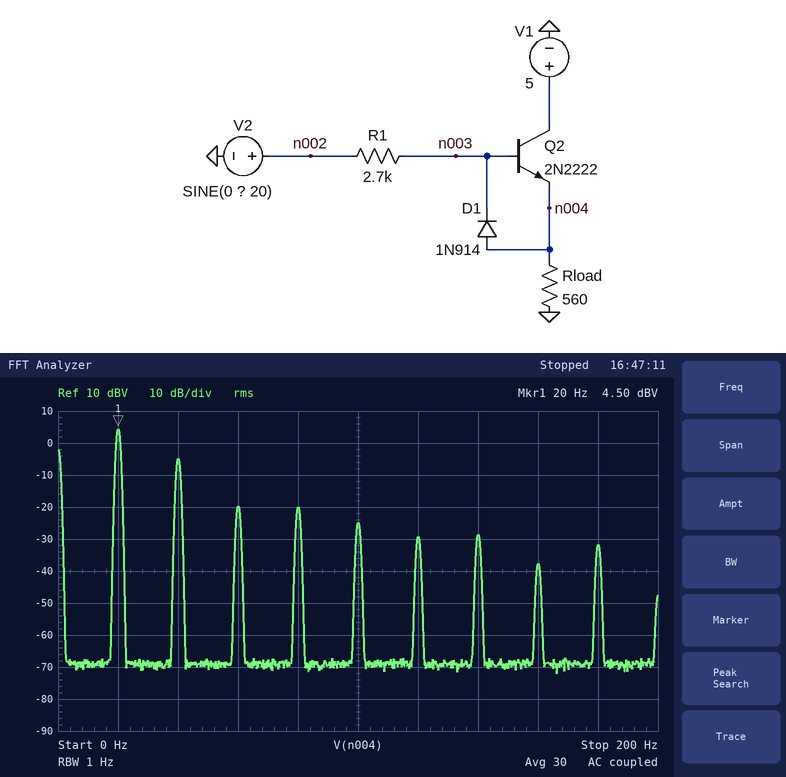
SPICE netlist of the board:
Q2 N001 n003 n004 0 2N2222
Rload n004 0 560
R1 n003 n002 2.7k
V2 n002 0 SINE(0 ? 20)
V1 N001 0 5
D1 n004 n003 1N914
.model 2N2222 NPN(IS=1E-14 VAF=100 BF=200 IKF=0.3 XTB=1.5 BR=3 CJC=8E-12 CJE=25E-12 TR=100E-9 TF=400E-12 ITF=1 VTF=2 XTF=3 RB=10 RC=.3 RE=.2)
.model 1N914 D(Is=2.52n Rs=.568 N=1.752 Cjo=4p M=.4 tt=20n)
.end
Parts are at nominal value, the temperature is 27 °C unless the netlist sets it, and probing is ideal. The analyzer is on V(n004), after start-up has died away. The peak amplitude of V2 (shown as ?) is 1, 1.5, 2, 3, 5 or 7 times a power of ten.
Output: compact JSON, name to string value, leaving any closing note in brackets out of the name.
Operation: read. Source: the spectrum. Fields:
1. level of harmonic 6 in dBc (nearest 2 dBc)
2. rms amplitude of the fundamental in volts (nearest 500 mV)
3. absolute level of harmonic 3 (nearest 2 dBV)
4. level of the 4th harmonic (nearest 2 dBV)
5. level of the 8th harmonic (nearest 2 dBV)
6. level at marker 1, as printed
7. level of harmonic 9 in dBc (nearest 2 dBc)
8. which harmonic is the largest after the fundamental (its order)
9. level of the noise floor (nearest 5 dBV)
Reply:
{"level of harmonic 6 in dBc": "-34 dBc", "rms amplitude of the fundamental in volts": "1.5 V", "absolute level of harmonic 3": "-20 dBV", "level of the 4th harmonic": "-20 dBV", "level of the 8th harmonic": "-38 dBV", "level at marker 1, as printed": "4.50 dBV", "level of harmonic 9 in dBc": "-36 dBc", "which harmonic is the largest after the fundamental": "2", "level of the noise floor": "-70 dBV"}
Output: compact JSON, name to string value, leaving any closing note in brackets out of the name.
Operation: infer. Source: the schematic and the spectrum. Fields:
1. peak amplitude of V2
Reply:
{"peak amplitude of V2": "5 V"}
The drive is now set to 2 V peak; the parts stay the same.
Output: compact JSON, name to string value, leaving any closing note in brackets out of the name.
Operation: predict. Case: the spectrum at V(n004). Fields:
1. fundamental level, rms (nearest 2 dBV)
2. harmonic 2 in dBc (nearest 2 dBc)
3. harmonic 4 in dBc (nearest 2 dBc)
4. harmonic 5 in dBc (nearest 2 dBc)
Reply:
{"fundamental level, rms": "-6 dBV", "harmonic 2 in dBc": "-8 dBc", "harmonic 4 in dBc": "-32 dBc", "harmonic 5 in dBc": "-22 dBc"}
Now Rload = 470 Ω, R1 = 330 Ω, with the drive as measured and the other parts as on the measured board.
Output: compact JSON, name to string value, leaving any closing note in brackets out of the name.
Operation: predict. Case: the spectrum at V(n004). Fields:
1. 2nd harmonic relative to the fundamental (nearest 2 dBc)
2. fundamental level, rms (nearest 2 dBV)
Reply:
{"2nd harmonic relative to the fundamental": "-18 dBc", "fundamental level, rms": "8 dBV"}
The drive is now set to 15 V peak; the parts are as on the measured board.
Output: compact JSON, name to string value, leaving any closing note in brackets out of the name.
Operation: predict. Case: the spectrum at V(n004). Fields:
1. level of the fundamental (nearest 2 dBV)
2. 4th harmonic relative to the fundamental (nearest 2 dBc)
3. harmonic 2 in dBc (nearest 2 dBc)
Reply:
{"level of the fundamental": "10 dBV", "4th harmonic relative to the fundamental": "-20 dBc", "harmonic 2 in dBc": "-32 dBc"}
